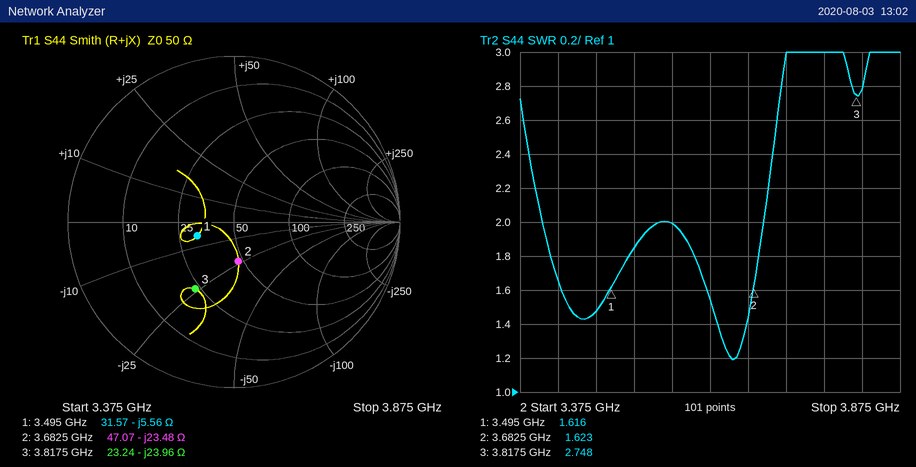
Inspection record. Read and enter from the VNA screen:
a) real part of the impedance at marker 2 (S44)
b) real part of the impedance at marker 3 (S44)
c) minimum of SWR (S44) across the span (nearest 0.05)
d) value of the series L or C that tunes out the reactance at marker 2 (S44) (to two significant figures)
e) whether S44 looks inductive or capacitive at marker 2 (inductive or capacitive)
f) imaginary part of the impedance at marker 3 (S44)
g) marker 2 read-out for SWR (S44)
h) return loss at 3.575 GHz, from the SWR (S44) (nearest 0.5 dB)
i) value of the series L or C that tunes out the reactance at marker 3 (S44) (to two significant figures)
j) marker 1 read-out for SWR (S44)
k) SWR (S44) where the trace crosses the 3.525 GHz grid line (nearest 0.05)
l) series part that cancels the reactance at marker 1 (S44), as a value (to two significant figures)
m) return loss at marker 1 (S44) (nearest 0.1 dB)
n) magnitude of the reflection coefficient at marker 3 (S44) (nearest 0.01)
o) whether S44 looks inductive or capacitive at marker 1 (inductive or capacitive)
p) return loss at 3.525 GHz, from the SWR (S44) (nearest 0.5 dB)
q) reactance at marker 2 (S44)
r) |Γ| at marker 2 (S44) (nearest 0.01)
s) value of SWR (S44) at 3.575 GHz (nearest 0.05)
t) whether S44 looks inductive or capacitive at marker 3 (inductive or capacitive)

47.07 Ω
23.24 Ω
1.20
1.0 nH
capacitive
-23.96 Ω
1.623
9.5 dB
1.00 nH
1.616
1.85
250 pH
12.6 dB
0.47
capacitive
10.5 dB
-23.48 Ω
0.24
2.00
capacitive
